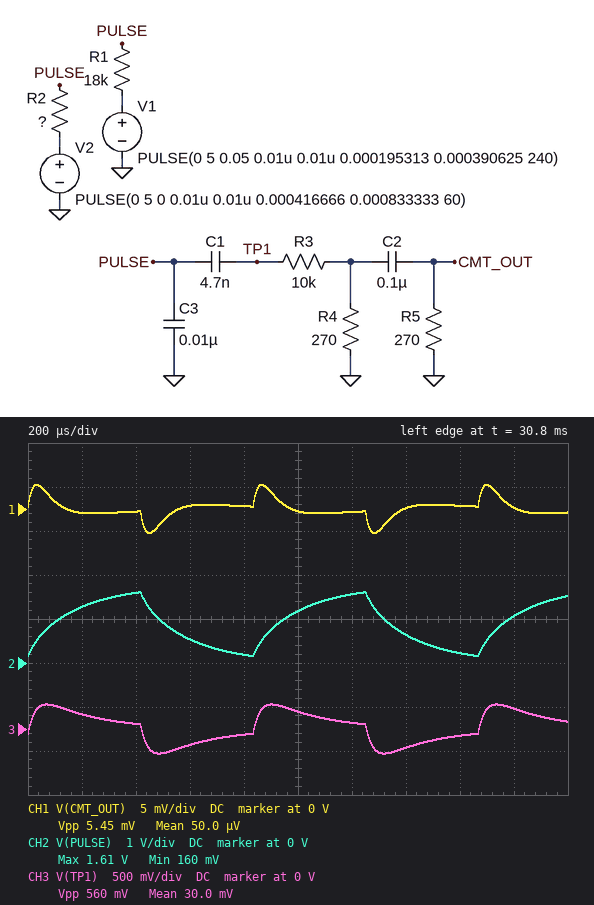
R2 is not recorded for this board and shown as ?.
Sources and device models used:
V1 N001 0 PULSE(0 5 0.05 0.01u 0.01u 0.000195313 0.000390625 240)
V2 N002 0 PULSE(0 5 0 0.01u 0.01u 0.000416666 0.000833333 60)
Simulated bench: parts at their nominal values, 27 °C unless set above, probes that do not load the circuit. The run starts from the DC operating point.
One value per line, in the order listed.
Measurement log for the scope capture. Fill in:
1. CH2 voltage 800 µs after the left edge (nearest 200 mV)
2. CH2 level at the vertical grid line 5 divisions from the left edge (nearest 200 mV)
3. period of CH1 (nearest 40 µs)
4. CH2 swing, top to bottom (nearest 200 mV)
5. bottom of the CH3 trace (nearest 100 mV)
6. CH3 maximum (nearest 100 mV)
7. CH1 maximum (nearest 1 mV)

200 mV
1.2 V
840 µs
1.4 V
-300 mV
300 mV
3 mV
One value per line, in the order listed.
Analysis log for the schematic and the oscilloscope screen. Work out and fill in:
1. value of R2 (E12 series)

33 kΩ
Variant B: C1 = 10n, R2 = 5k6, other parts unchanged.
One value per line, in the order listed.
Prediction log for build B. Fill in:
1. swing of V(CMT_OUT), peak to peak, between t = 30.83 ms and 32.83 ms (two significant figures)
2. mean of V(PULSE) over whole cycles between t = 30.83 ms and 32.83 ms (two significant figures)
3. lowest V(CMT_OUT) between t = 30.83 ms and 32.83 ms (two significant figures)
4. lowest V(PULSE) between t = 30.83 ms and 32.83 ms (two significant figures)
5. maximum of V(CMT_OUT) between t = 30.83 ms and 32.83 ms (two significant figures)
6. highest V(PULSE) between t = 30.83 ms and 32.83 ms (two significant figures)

30 mV
1.9 V
-15 mV
120 mV
15 mV
3.7 V
